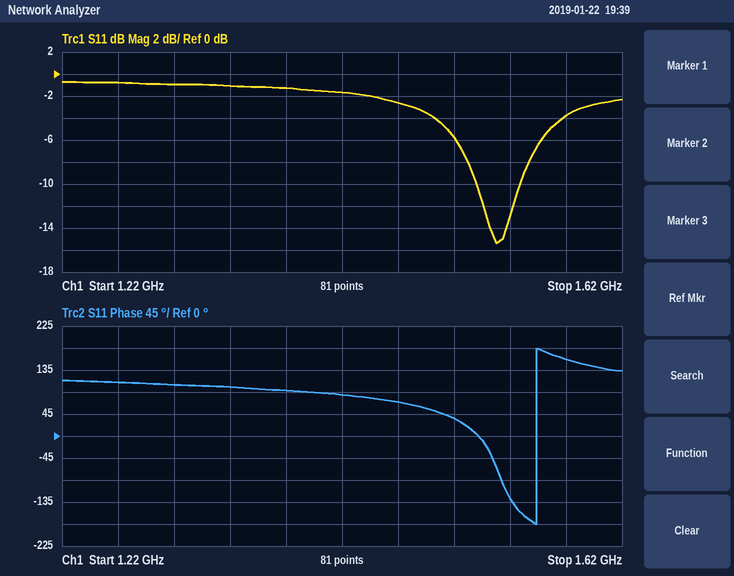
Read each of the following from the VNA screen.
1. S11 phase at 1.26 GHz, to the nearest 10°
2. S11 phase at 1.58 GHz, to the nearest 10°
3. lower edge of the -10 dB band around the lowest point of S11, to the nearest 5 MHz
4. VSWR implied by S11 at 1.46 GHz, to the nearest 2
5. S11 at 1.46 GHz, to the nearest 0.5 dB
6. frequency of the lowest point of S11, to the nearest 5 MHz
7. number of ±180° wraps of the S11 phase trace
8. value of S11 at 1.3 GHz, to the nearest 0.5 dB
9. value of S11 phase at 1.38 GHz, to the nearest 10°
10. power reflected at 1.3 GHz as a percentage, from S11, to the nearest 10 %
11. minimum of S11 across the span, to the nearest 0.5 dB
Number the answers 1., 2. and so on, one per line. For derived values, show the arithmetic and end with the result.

1. 110°
2. 160°
3. 1.515 GHz
4. |Γ| = 10^(-2.5/20) = 0.7499; VSWR = (1 + 0.7499)/(1 − 0.7499) ≈ 7.00, so 6 to the nearest 2
5. -2.5 dB
6. 1.530 GHz
7. 1
8. -1.0 dB
9. 90°
10. 10^(-1/10) ≈ 79.4 %, so 80 % to the nearest 10 %
11. -15.5 dB
